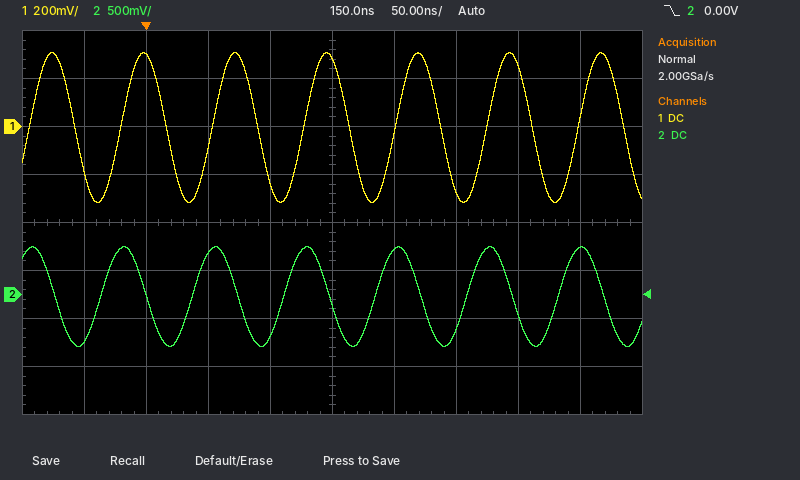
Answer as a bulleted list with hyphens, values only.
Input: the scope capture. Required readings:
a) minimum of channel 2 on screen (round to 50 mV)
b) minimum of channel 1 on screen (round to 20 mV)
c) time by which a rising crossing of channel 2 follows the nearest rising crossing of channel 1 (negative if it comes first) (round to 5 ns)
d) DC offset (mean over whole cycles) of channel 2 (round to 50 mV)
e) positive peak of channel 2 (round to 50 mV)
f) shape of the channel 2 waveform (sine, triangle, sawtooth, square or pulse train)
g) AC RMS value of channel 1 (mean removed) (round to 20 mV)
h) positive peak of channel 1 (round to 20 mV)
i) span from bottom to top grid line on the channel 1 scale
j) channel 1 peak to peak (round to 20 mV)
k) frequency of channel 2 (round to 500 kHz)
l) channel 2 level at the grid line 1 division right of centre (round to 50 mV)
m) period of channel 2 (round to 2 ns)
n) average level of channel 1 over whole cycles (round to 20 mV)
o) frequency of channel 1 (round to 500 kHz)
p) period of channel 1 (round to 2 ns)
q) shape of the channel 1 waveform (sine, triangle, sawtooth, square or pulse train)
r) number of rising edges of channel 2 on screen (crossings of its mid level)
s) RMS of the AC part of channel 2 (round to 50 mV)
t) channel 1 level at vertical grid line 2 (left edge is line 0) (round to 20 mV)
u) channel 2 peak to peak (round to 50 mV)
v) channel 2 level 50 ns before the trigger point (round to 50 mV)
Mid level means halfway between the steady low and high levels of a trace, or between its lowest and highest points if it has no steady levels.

- -550 mV
- -320 mV
- -15 ns
- 0 mV
- 500 mV
- sine
- 220 mV
- 300 mV
- 1.6 V
- 620 mV
- 13.5 MHz
- 450 mV
- 74 ns
- 0 mV
- 13.5 MHz
- 74 ns
- sine
- 6
- 350 mV
- 300 mV
- 1.05 V
- -500 mV
